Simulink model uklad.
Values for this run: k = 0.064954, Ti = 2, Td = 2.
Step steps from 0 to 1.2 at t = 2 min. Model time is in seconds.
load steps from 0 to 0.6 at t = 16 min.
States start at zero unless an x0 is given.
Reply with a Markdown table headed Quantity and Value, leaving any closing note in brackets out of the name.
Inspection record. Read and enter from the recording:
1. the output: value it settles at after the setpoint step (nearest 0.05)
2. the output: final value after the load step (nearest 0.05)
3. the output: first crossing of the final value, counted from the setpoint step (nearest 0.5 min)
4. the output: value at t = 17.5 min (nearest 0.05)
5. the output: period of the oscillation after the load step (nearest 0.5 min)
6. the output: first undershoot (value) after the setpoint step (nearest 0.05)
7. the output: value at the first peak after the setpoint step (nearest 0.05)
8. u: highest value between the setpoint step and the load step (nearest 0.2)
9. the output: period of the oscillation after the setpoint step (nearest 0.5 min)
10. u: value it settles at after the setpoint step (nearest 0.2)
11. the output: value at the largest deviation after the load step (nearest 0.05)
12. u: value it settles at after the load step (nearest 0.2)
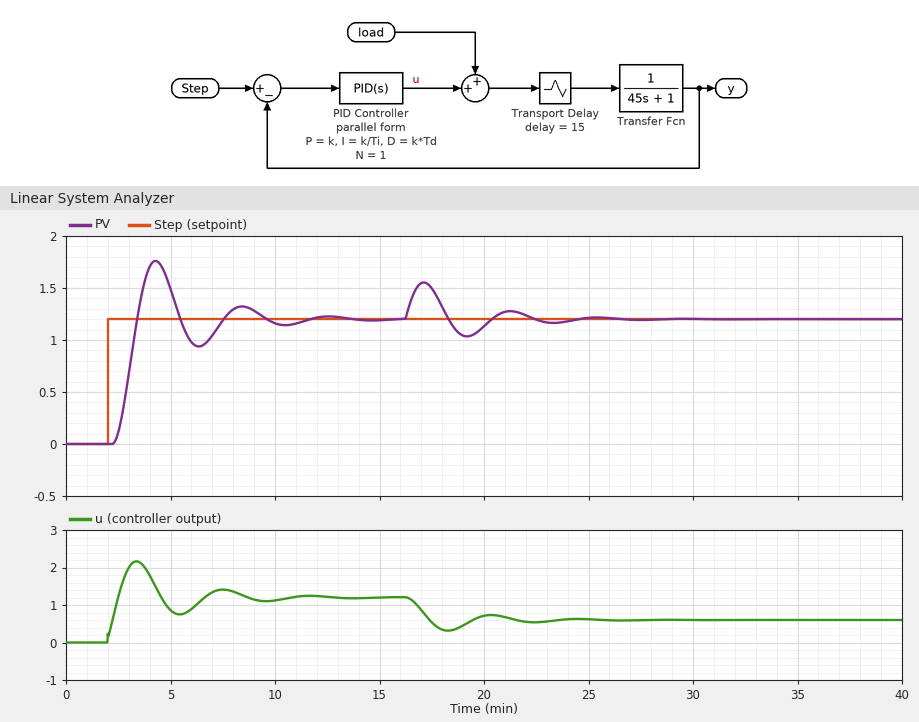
| Quantity | Value |
|---|---|
| the output: value it settles at after the setpoint step | 1.20 |
| the output: final value after the load step | 1.20 |
| the output: first crossing of the final value, counted from the setpoint step | 1.5 min |
| the output: value at t = 17.5 min | 1.50 |
| the output: period of the oscillation after the load step | 4.0 min |
| the output: first undershoot (value) after the setpoint step | 0.95 |
| the output: value at the first peak after the setpoint step | 1.75 |
| u: highest value between the setpoint step and the load step | 2.2 |
| the output: period of the oscillation after the setpoint step | 4.0 min |
| u: value it settles at after the setpoint step | 1.2 |
| the output: value at the largest deviation after the load step | 1.55 |
| u: value it settles at after the load step | 0.6 |
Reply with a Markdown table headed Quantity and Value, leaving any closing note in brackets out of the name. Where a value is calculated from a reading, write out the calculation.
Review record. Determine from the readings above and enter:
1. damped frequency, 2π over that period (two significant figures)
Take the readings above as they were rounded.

| Quantity | Value |
|---|---|
| damped frequency, 2π over that period | 2π / 4 = 1.6 rad/min |
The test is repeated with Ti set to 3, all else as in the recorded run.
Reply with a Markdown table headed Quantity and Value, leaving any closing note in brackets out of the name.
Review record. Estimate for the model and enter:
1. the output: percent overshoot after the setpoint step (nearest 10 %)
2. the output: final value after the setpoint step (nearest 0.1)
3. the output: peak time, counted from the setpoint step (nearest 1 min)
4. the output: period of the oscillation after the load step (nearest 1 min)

| Quantity | Value |
|---|---|
| the output: percent overshoot after the setpoint step | 30 % |
| the output: final value after the setpoint step | 1.2 |
| the output: peak time, counted from the setpoint step | 3 min |
| the output: period of the oscillation after the load step | 5 min |
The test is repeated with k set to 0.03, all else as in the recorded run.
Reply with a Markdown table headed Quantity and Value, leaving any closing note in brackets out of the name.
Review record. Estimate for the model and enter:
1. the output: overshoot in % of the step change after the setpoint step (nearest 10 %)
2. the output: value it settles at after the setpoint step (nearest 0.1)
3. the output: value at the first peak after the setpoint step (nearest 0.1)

| Quantity | Value |
|---|---|
| the output: overshoot in % of the step change after the setpoint step | 20 % |
| the output: value it settles at after the setpoint step | 1.2 |
| the output: value at the first peak after the setpoint step | 1.4 |
